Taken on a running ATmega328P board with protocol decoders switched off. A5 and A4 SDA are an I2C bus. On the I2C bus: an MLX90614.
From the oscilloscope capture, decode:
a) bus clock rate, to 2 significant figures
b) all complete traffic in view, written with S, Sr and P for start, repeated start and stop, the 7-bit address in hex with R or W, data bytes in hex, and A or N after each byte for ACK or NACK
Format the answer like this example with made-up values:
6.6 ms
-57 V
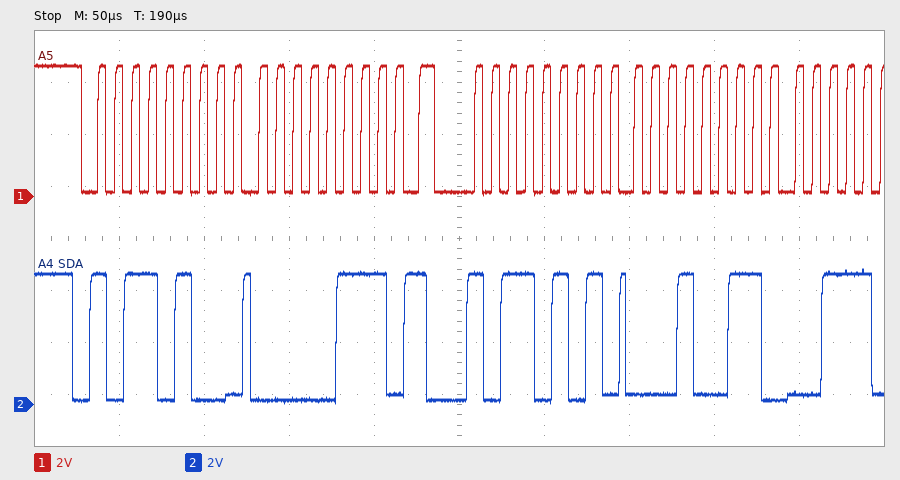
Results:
100 kHz
S 5AW A 07 A Sr 5AR A 13 A
